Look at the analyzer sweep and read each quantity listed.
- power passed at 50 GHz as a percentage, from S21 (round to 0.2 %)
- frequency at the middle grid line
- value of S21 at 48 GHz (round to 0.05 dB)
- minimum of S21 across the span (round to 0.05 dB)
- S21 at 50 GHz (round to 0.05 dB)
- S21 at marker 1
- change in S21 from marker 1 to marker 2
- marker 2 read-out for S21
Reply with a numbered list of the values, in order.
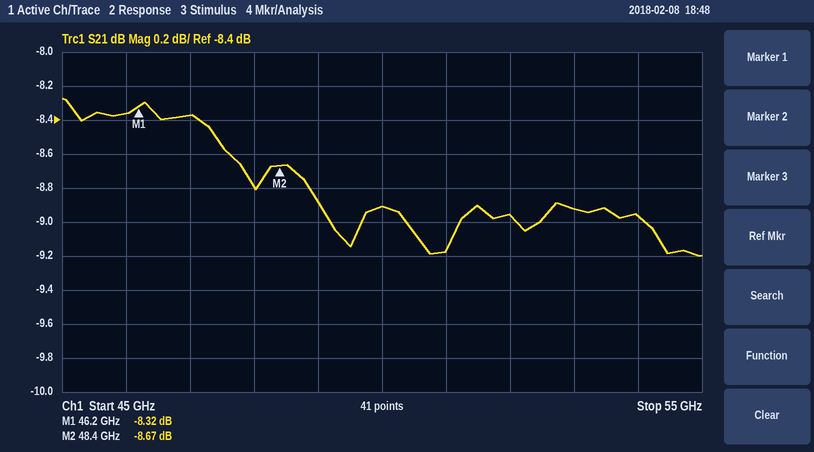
1. 12.8 %
2. 50 GHz
3. -8.80 dB
4. -9.20 dB
5. -8.90 dB
6. -8.32 dB
7. -0.35 dB
8. -8.67 dB
